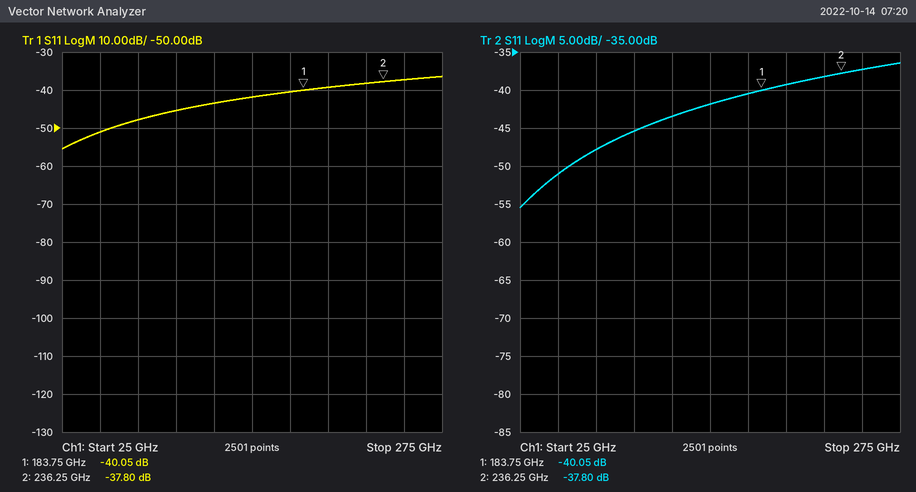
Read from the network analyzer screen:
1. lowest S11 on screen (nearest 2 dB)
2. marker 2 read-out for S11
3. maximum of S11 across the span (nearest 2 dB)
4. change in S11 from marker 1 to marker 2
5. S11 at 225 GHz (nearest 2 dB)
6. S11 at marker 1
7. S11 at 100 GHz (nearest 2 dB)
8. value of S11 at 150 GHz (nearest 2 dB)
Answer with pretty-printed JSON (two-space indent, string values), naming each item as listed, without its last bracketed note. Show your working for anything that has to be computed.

{
  "lowest S11 on screen": "-56 dB",
  "marker 2 read-out for S11": "-37.80 dB",
  "maximum of S11 across the span": "-36 dB",
  "change in S11 from marker 1 to marker 2": "-37.8 − (-40.05) = 2.25 dB",
  "S11 at 225 GHz": "-38 dB",
  "S11 at marker 1": "-40.05 dB",
  "S11 at 100 GHz": "-46 dB",
  "value of S11 at 150 GHz": "-42 dB"
}
